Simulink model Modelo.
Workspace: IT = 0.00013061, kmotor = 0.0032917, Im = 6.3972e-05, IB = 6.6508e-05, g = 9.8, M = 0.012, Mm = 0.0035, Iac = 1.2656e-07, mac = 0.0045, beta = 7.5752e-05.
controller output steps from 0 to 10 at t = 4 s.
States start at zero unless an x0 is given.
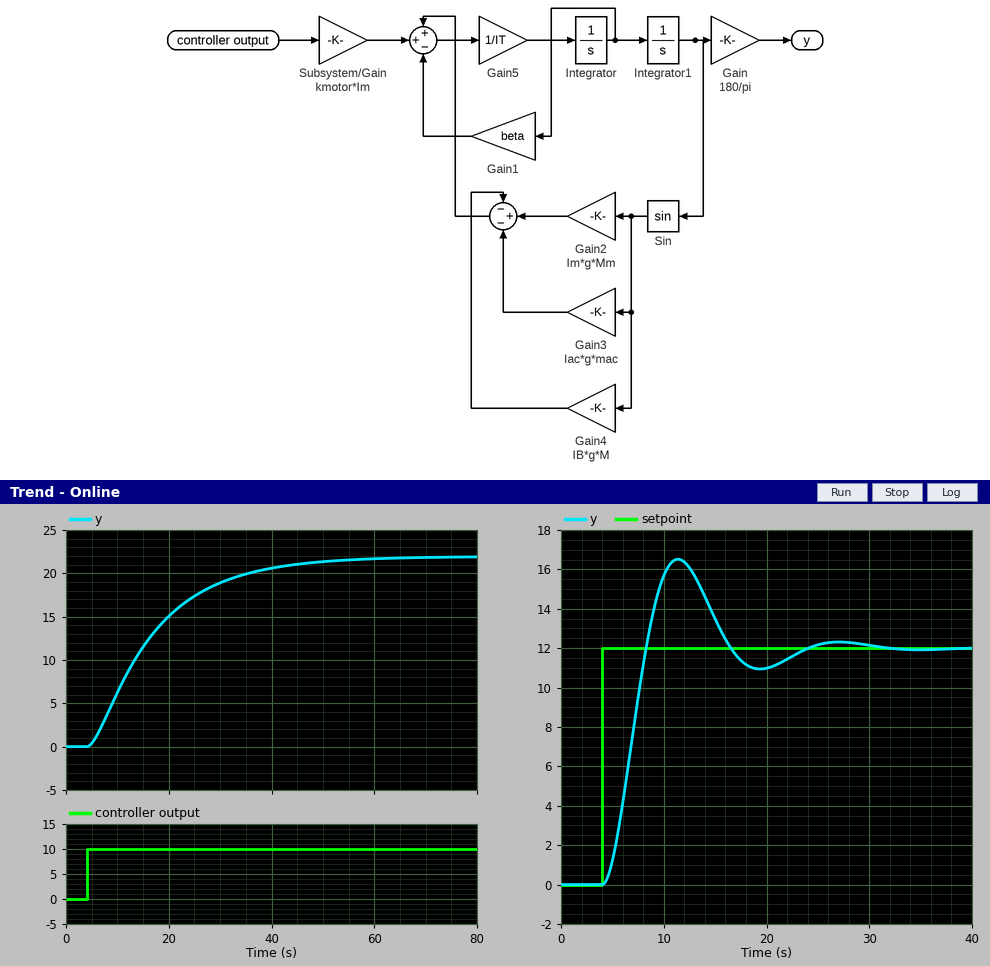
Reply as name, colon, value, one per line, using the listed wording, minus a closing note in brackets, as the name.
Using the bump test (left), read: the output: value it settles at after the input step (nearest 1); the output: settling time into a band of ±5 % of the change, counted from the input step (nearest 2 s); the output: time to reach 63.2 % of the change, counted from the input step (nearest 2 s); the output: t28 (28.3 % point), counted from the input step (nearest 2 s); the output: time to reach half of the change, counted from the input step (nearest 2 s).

the output: value it settles at after the input step: 22
the output: settling time into a band of ±5 % of the change, counted from the input step: 38 s
the output: time to reach 63.2 % of the change, counted from the input step: 14 s
the output: t28 (28.3 % point), counted from the input step: 6 s
the output: time to reach half of the change, counted from the input step: 10 s
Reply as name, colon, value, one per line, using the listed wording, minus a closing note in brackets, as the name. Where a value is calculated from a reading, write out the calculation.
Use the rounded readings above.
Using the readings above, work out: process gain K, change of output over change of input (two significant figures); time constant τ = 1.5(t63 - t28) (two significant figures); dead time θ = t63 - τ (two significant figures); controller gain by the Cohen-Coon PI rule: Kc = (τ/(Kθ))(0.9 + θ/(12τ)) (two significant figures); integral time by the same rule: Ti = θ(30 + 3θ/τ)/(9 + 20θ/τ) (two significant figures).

process gain K, change of output over change of input: (22 - 0) / 10 = 2.2
time constant τ = 1.5(t63 - t28): 1.5 × (14 - 6) = 12 s
dead time θ = t63 - τ: 14 - 12 = 2.0 s
controller gain by the Cohen-Coon PI rule: Kc = (τ/(Kθ))(0.9 + θ/(12τ)): 12 / (2.2 × 2) × (0.9 + 2 / (12 × 12)) = 2.5
integral time by the same rule: Ti = θ(30 + 3θ/τ)/(9 + 20θ/τ): 2 × (30 + 3 × 2 / 12) / (9 + 20 × 2 / 12) = 4.9 s
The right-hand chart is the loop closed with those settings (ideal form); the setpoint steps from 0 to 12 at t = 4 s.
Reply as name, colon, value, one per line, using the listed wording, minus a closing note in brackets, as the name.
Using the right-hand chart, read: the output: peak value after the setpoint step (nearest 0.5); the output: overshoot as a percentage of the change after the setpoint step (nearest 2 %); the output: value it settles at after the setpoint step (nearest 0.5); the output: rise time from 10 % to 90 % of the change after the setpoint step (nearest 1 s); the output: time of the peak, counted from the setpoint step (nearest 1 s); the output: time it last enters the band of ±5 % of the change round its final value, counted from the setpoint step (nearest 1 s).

the output: peak value after the setpoint step: 16.5
the output: overshoot as a percentage of the change after the setpoint step: 38 %
the output: value it settles at after the setpoint step: 12.0
the output: rise time from 10 % to 90 % of the change after the setpoint step: 3 s
the output: time of the peak, counted from the setpoint step: 7 s
the output: time it last enters the band of ±5 % of the change round its final value, counted from the setpoint step: 18 s
